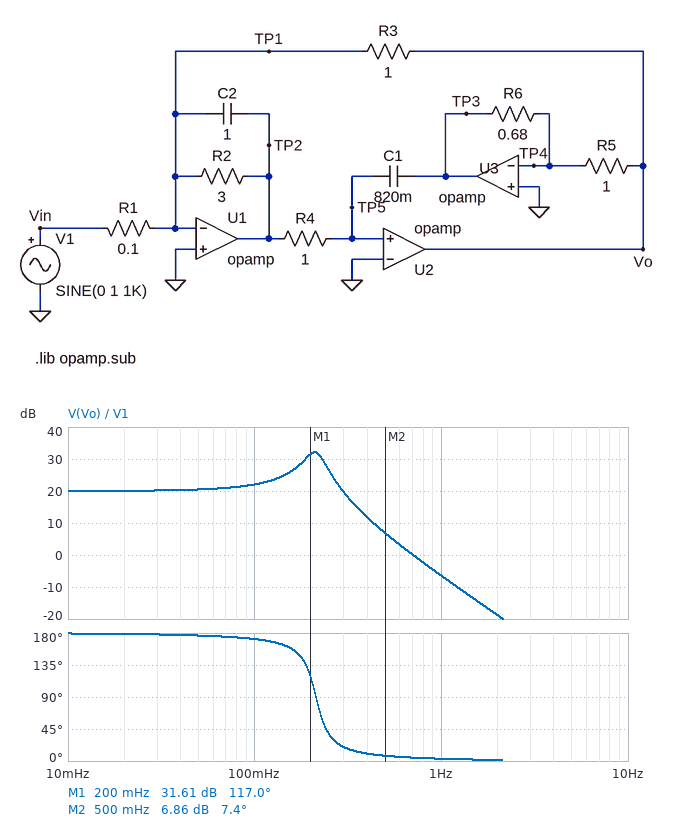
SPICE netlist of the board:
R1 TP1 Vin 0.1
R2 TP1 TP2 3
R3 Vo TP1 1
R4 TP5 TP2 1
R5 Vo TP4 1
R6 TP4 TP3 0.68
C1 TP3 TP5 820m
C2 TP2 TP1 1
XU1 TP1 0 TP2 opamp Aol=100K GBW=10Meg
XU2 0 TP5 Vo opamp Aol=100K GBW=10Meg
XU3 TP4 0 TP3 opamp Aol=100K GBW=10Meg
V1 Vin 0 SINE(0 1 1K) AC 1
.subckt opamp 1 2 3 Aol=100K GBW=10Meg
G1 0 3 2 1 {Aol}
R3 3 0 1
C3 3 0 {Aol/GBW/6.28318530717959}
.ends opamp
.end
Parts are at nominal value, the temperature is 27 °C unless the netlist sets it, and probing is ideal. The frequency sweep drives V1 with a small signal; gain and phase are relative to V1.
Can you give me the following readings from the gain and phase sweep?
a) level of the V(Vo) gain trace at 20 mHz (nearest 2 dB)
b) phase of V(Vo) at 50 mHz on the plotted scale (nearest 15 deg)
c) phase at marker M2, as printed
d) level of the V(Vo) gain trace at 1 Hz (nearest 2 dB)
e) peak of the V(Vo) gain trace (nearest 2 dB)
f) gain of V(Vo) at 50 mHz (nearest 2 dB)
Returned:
20 dB
180 deg
7.4 deg
-6 dB
32 dB
20 dB
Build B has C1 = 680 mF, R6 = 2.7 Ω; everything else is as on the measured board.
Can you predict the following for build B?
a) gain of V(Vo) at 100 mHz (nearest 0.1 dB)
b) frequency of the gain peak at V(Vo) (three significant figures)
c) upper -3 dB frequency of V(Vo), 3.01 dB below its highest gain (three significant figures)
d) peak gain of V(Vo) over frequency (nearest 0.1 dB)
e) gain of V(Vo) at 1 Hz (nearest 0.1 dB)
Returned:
26.5 dB
111 mHz
136 mHz
27.1 dB
-17.1 dB
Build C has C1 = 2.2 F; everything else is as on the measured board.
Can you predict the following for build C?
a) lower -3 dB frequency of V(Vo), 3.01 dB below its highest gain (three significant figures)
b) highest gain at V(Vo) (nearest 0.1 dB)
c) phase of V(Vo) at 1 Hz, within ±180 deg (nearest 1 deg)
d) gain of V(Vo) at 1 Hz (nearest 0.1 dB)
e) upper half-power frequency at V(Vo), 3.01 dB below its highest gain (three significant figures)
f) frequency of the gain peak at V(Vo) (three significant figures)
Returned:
93.6 mHz
28.0 dB
3 deg
-15.3 dB
149 mHz
125 mHz
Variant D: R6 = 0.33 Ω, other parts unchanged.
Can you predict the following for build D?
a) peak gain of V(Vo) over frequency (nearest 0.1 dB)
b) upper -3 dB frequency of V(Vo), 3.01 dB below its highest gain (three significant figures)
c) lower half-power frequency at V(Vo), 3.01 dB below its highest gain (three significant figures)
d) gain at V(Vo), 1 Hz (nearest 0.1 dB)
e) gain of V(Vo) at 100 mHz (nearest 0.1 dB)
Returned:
35.2 dB
329 mHz
276 mHz
0.3 dB
21.0 dB
